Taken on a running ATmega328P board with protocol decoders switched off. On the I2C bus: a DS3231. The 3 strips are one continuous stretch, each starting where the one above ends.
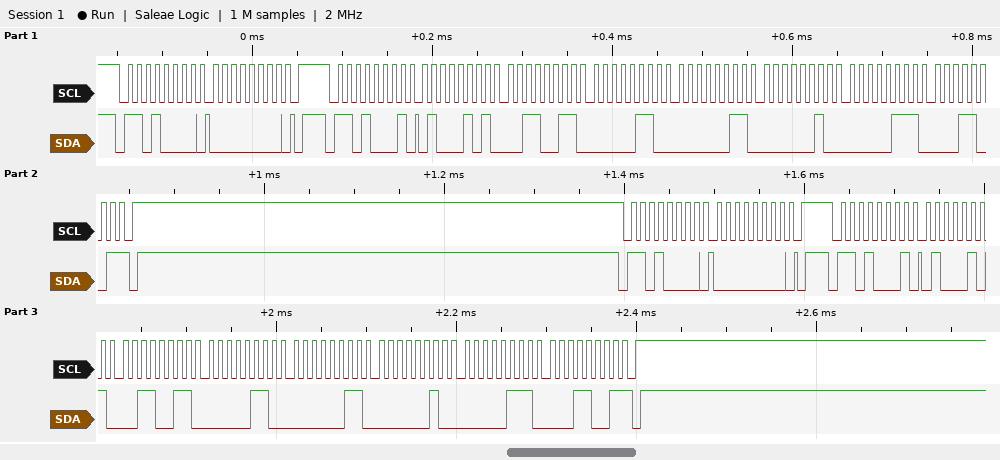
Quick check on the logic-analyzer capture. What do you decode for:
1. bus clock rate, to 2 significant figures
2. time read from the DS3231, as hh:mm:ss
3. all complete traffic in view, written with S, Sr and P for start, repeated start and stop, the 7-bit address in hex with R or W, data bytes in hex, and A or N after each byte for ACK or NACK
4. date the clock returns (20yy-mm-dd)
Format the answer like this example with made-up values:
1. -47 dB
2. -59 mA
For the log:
1. 100 kHz
2. 06:33:45
3. S 68W A 00 A P S 68R A 45 A 33 A 06 A 03 A 02 A 07 A 19 N P S 68W A 00 A P S 68R A 45 A 33 A 06 A 03 A 02 A 07 A 19 N P
4. 2019-07-02
